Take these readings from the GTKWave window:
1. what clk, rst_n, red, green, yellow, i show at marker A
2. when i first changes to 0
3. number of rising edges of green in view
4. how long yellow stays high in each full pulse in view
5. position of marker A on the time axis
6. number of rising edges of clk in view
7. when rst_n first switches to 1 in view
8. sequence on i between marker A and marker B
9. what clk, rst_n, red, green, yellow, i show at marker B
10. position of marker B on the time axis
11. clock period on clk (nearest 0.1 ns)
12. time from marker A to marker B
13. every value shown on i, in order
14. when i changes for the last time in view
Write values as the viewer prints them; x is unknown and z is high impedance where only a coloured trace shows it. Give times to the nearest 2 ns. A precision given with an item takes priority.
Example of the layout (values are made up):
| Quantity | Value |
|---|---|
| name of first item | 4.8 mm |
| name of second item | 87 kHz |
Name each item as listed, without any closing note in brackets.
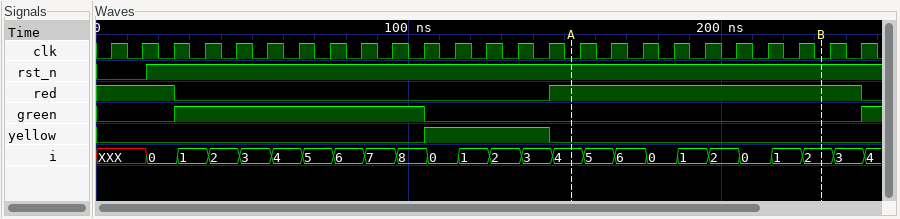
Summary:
| Quantity | Value |
|---|---|
| what clk, rst_n, red, green, yellow, i show at marker A | clk=0, rst_n=1, red=1, green=0, yellow=0, i=4 |
| when i first changes to 0 | 16 ns |
| number of rising edges of green in view | 2 |
| how long yellow stays high in each full pulse in view | 40 ns |
| position of marker A on the time axis | 152 ns |
| number of rising edges of clk in view | 25 |
| when rst_n first switches to 1 in view | 16 ns |
| sequence on i between marker A and marker B | 4, 5, 6, 0, 1, 2, 0, 1, 2 |
| what clk, rst_n, red, green, yellow, i show at marker B | clk=0, rst_n=1, red=1, green=0, yellow=0, i=2 |
| position of marker B on the time axis | 232 ns |
| clock period on clk | 10 ns |
| time from marker A to marker B | 80 ns |
| every value shown on i, in order | XXX, 0, 1, 2, 3, 4, 5, 6, 7, 8, 0, 1, 2, 3, 4, 5, 6, 0, 1, 2, 0, 1, 2, 3, 4 |
| when i changes for the last time in view | 246 ns |
